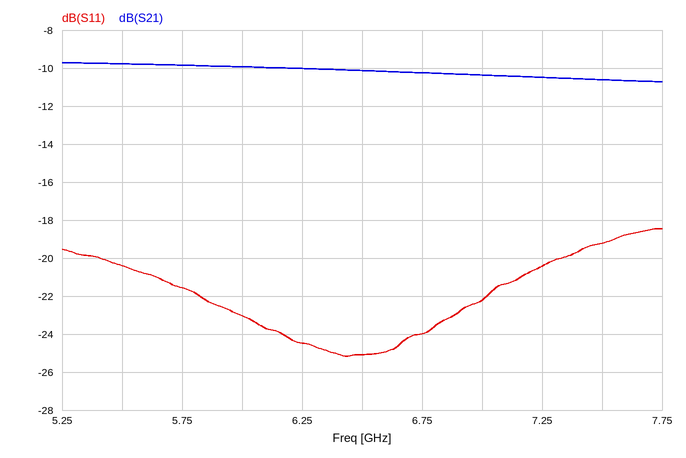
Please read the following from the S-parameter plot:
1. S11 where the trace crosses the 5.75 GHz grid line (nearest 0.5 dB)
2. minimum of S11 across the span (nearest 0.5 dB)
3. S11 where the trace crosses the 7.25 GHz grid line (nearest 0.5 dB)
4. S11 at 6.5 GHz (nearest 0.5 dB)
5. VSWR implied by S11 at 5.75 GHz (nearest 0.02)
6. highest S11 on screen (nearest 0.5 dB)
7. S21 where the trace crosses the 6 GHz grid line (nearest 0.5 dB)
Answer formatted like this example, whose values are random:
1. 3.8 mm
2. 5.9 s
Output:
1. -21.5 dB
2. -25.0 dB
3. -20.5 dB
4. -25.0 dB
5. 1.18
6. -18.5 dB
7. -10.0 dB
